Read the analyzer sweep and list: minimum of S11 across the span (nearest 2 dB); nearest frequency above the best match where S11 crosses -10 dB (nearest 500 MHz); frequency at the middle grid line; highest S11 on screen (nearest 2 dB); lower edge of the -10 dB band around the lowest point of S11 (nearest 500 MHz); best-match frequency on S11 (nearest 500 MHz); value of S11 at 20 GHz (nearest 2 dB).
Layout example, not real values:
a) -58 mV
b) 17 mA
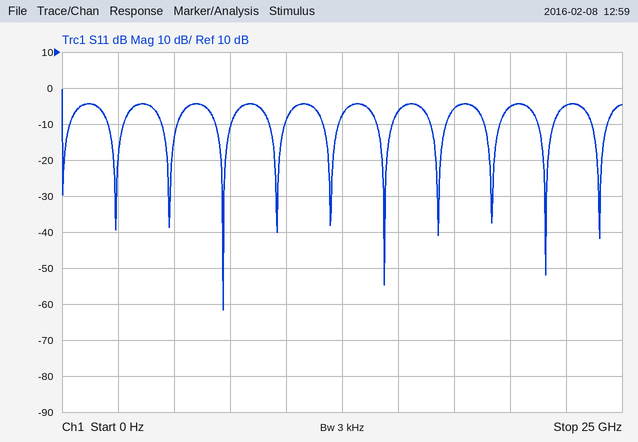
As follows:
a) -62 dB
b) 7.5 GHz
c) 12.5 GHz
d) 0 dB
e) 7.0 GHz
f) 7.0 GHz
g) -6 dB
